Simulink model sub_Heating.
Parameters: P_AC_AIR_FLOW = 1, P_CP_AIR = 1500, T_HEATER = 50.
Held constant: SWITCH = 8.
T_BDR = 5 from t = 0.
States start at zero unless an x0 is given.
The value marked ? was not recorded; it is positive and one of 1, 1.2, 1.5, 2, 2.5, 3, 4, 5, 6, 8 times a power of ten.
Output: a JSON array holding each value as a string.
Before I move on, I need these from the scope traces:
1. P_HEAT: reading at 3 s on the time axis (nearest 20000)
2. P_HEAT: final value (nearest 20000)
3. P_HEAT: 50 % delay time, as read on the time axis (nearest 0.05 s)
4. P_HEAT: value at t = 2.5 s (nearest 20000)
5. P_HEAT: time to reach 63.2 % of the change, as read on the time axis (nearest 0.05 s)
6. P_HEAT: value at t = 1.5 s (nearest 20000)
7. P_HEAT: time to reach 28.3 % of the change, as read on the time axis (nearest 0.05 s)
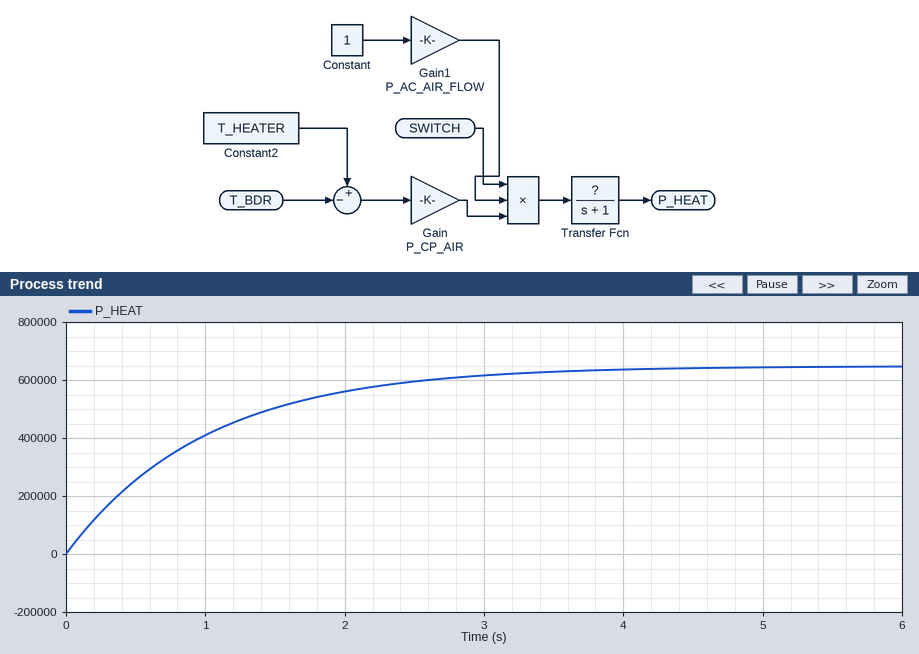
["620000", "640000", "0.70 s", "600000", "1.00 s", "500000", "0.35 s"]
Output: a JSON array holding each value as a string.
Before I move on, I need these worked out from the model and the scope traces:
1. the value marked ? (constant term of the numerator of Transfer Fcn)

["1.2"]
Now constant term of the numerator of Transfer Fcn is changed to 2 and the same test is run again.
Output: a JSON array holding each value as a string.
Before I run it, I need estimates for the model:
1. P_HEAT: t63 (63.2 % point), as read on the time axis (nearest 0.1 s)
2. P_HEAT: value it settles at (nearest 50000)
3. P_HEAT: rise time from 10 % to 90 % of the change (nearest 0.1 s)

["1.0 s", "1100000", "2.2 s"]
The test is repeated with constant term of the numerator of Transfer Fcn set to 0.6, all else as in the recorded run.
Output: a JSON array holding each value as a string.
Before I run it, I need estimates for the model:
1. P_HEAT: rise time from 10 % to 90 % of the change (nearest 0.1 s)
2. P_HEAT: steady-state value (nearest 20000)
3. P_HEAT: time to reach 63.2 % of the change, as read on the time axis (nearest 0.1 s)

["2.2 s", "320000", "1.0 s"]
